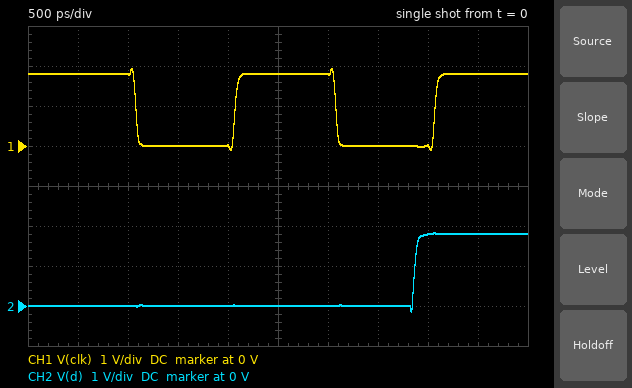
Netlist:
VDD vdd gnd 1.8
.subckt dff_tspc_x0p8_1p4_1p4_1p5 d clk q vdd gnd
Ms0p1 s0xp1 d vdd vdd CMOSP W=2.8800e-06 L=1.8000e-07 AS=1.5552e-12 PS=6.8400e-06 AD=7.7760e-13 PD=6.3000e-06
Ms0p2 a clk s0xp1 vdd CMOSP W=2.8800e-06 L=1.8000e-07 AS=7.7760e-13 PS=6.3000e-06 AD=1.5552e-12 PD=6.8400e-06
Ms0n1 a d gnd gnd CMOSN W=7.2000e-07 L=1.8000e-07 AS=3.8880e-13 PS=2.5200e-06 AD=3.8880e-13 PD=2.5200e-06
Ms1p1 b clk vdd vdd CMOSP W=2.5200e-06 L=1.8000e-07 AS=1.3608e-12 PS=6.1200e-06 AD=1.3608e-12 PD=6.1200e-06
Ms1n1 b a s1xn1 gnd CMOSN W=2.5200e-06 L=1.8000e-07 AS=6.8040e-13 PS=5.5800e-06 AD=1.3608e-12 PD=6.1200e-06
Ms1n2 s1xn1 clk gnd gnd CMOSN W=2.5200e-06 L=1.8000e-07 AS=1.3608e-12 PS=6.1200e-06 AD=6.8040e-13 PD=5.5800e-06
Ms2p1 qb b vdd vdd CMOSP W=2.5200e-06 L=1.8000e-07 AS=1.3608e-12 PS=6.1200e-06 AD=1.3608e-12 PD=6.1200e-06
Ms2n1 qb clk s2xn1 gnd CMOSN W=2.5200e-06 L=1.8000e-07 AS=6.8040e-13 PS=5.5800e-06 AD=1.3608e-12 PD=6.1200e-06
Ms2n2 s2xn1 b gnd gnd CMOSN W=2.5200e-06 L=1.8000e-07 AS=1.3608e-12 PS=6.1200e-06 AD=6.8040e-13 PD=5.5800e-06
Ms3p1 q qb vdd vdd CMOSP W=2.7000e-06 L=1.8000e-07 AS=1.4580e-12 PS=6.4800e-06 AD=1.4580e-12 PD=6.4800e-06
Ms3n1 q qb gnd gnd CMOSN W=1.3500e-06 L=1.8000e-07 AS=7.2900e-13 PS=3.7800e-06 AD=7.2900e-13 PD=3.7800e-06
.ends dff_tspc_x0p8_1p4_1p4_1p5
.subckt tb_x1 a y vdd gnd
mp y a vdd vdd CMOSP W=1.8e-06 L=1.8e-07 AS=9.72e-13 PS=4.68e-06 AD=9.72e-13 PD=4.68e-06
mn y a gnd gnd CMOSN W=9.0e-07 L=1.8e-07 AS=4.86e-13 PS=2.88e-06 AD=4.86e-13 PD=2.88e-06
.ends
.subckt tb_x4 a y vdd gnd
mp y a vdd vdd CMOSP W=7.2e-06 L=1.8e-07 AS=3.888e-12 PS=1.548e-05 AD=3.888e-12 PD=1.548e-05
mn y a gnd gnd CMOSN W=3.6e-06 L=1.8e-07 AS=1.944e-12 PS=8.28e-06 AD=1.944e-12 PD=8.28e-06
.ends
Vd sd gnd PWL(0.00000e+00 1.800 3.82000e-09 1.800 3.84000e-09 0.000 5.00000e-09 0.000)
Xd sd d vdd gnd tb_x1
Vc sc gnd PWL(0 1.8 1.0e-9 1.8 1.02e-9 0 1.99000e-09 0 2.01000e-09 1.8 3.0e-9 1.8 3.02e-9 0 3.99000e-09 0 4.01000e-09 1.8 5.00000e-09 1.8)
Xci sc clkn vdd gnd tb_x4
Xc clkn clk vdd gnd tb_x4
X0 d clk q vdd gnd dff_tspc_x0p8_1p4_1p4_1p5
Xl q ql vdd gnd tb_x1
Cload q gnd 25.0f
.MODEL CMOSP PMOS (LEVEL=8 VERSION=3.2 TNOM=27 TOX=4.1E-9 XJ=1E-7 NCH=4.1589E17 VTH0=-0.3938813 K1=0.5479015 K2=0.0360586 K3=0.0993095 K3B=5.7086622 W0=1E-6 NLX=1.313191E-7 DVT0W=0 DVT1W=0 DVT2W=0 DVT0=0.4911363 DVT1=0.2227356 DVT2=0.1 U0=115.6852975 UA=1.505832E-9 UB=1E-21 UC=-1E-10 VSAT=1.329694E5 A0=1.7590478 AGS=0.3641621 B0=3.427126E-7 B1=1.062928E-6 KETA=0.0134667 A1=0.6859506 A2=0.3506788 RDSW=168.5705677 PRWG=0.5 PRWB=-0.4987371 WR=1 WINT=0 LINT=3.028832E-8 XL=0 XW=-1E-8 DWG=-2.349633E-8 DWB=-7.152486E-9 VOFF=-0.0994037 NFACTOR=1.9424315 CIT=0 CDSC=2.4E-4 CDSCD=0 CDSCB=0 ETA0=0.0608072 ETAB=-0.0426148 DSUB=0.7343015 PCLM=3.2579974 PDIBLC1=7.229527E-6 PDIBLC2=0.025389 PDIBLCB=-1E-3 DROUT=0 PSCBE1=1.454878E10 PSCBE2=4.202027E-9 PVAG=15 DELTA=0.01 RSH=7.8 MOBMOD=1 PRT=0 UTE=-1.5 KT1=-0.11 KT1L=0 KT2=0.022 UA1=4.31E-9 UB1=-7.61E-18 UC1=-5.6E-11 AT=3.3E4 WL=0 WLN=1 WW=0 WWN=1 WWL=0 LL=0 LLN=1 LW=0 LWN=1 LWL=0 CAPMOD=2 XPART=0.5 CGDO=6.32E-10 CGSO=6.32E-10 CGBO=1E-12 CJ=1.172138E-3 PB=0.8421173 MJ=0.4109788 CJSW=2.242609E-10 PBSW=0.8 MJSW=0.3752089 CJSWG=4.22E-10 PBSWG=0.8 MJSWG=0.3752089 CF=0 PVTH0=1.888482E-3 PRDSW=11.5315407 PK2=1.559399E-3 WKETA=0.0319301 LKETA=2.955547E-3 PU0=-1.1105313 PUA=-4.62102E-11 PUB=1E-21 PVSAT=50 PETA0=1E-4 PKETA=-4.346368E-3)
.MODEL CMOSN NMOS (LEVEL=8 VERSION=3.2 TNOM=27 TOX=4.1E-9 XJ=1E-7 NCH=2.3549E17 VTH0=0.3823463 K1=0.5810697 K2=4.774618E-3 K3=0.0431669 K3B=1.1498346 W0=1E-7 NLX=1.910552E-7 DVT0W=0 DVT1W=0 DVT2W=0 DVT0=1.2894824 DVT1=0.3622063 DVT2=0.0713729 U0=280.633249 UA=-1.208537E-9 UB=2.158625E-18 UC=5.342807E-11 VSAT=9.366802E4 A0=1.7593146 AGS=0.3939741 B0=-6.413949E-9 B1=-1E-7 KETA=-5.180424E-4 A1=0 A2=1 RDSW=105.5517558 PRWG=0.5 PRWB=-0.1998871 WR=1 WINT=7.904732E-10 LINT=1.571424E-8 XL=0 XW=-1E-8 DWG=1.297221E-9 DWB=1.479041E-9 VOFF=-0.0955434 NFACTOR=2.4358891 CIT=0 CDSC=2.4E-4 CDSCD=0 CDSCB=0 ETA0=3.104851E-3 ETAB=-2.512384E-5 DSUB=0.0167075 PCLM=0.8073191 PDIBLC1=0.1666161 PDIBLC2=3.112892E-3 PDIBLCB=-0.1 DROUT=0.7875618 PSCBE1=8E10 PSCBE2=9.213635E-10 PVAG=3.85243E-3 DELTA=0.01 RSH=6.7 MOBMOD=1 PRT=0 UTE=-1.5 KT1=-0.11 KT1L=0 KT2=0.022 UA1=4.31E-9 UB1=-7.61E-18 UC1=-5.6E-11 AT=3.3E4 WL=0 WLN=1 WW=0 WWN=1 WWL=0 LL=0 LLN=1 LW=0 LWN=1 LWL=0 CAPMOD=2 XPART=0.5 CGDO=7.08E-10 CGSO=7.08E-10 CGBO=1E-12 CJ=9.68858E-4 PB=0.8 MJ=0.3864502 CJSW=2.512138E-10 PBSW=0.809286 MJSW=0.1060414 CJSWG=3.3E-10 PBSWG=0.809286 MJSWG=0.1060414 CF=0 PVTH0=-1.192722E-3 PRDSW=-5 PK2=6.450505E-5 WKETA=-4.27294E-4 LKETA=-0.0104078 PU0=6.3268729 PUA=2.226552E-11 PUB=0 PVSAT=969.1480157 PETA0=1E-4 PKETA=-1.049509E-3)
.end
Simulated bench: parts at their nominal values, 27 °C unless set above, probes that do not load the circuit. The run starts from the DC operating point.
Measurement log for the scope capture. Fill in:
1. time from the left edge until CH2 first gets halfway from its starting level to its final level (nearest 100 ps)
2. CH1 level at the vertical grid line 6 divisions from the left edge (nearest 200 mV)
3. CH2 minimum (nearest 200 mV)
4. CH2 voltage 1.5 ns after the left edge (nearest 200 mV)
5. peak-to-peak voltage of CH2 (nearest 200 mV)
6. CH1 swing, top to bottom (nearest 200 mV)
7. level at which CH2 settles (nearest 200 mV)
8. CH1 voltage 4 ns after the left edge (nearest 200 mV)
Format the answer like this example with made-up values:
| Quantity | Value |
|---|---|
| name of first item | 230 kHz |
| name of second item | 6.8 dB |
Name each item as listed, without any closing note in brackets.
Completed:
| Quantity | Value |
|---|---|
| time from the left edge until CH2 first gets halfway from its starting level to its final level | 3.9 ns |
| CH1 level at the vertical grid line 6 divisions from the left edge | 1.8 V |
| CH2 minimum | -200 mV |
| CH2 voltage 1.5 ns after the left edge | 0 V |
| peak-to-peak voltage of CH2 | 2.0 V |
| CH1 swing, top to bottom | 2.0 V |
| level at which CH2 settles | 1.8 V |
| CH1 voltage 4 ns after the left edge | 0 V |
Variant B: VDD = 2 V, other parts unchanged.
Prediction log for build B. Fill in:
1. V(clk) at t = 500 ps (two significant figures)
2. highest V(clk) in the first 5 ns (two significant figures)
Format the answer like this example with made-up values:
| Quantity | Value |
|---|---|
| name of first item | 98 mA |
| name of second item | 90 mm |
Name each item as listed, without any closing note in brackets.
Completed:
| Quantity | Value |
|---|---|
| V(clk) at t = 500 ps | 2.0 V |
| highest V(clk) in the first 5 ns | 2.1 V |
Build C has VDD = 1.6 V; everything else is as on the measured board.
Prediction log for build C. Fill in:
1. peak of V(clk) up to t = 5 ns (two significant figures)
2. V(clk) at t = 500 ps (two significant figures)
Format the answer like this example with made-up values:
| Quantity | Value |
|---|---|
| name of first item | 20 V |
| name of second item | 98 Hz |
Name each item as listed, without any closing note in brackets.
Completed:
| Quantity | Value |
|---|---|
| peak of V(clk) up to t = 5 ns | 1.7 V |
| V(clk) at t = 500 ps | 1.6 V |
